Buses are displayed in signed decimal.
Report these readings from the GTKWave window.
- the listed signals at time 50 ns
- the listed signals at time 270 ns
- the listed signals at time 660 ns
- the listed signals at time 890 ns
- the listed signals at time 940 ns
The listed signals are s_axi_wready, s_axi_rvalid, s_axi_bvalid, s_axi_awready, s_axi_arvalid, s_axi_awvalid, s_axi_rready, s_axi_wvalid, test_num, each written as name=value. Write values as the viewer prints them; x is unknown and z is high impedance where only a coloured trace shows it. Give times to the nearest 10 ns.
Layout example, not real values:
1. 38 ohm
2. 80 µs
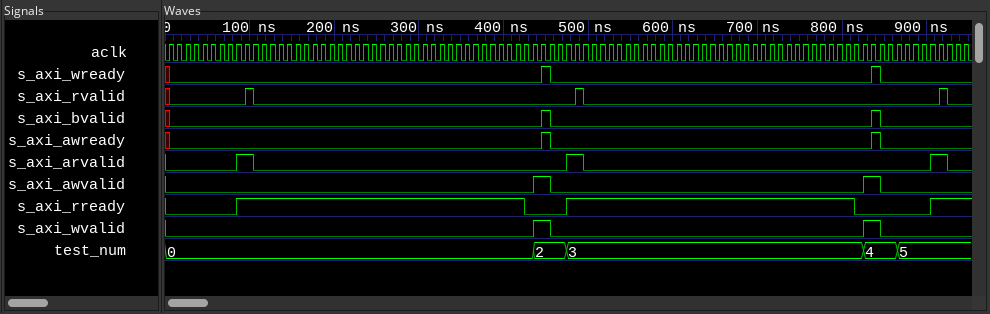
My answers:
1. s_axi_wready=0, s_axi_rvalid=0, s_axi_bvalid=0, s_axi_awready=0, s_axi_arvalid=0, s_axi_awvalid=0, s_axi_rready=0, s_axi_wvalid=0, test_num=0
2. s_axi_wready=0, s_axi_rvalid=0, s_axi_bvalid=0, s_axi_awready=0, s_axi_arvalid=0, s_axi_awvalid=0, s_axi_rready=1, s_axi_wvalid=0, test_num=0
3. s_axi_wready=0, s_axi_rvalid=0, s_axi_bvalid=0, s_axi_awready=0, s_axi_arvalid=0, s_axi_awvalid=0, s_axi_rready=1, s_axi_wvalid=0, test_num=3
4. s_axi_wready=0, s_axi_rvalid=0, s_axi_bvalid=0, s_axi_awready=0, s_axi_arvalid=0, s_axi_awvalid=0, s_axi_rready=0, s_axi_wvalid=0, test_num=5
5. s_axi_wready=0, s_axi_rvalid=0, s_axi_bvalid=0, s_axi_awready=0, s_axi_arvalid=0, s_axi_awvalid=0, s_axi_rready=1, s_axi_wvalid=0, test_num=5
